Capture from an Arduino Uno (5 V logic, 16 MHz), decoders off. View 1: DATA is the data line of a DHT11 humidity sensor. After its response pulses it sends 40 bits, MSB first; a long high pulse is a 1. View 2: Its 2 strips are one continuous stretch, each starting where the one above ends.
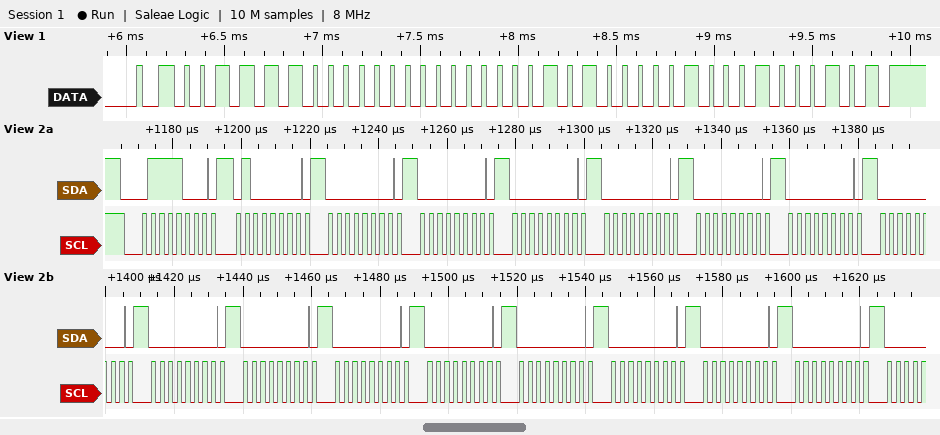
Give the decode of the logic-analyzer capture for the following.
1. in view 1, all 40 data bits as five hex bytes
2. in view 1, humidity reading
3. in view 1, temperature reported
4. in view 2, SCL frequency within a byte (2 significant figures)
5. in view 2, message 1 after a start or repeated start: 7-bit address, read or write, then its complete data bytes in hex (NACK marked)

3C 00 05 04 45
60 %
5.4 °C
400 kHz
0x3C write: 40 00 00 00 00 00 00 00 00 00 00 00 00 00 00 00
